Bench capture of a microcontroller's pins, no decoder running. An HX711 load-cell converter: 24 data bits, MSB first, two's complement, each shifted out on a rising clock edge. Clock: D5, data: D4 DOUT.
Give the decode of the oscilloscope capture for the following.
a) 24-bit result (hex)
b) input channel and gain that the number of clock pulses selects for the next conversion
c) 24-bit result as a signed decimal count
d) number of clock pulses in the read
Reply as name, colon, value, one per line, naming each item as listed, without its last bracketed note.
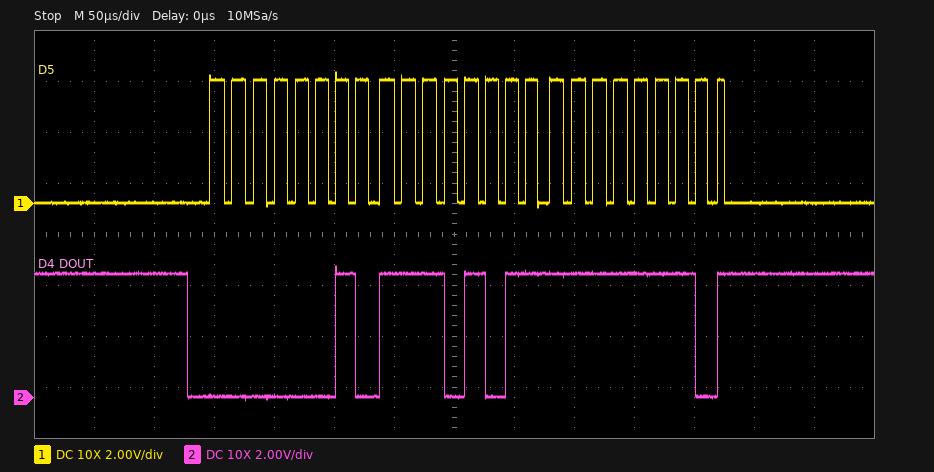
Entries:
24-bit result: 0x02EBFE
input channel and gain that the number of clock pulses selects for the next conversion: channel A, gain 128
24-bit result as a signed decimal count: 191486
number of clock pulses in the read: 25
